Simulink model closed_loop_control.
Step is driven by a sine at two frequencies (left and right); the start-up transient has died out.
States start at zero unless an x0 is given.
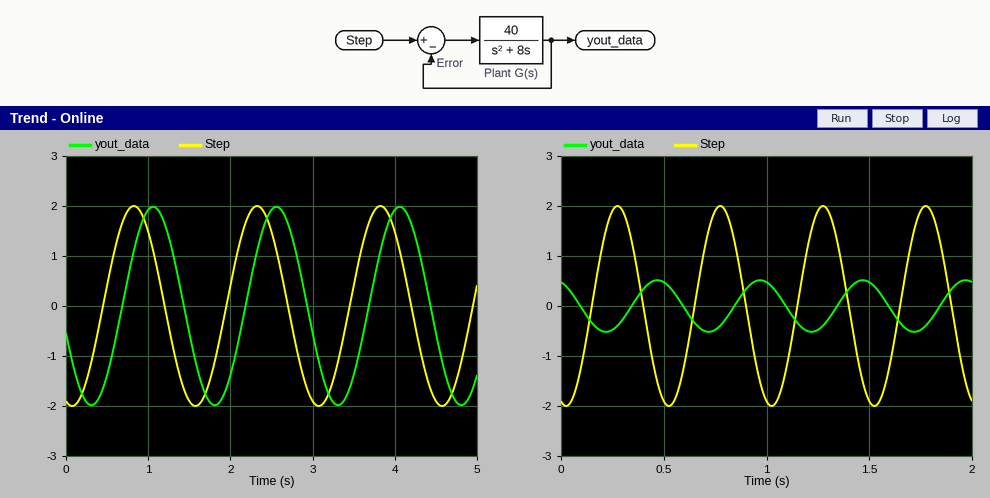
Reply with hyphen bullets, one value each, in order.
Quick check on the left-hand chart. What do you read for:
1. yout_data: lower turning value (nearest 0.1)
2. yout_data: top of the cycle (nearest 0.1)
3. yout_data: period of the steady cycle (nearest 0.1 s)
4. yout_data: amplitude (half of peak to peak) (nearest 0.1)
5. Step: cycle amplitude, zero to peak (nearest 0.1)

- -2.0
- 2.0
- 1.5 s
- 2.0
- 2.0
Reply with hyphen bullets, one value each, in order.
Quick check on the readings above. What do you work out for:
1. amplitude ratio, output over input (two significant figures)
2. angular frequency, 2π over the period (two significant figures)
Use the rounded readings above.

- 1.0
- 4.2 rad/s
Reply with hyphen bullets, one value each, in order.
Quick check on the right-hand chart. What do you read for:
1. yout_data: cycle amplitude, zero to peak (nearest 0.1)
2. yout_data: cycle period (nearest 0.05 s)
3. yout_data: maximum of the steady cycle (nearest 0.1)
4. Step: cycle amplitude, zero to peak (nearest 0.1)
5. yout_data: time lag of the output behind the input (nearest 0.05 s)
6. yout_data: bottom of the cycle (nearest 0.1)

- 0.5
- 0.50 s
- 0.5
- 2.0
- 0.20 s
- -0.5
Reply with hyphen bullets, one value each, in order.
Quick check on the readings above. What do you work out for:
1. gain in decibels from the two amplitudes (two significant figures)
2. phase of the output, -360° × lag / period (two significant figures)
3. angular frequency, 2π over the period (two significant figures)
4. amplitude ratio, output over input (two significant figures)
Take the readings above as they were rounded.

- -12 dB
- -140°
- 13 rad/s
- 0.25
